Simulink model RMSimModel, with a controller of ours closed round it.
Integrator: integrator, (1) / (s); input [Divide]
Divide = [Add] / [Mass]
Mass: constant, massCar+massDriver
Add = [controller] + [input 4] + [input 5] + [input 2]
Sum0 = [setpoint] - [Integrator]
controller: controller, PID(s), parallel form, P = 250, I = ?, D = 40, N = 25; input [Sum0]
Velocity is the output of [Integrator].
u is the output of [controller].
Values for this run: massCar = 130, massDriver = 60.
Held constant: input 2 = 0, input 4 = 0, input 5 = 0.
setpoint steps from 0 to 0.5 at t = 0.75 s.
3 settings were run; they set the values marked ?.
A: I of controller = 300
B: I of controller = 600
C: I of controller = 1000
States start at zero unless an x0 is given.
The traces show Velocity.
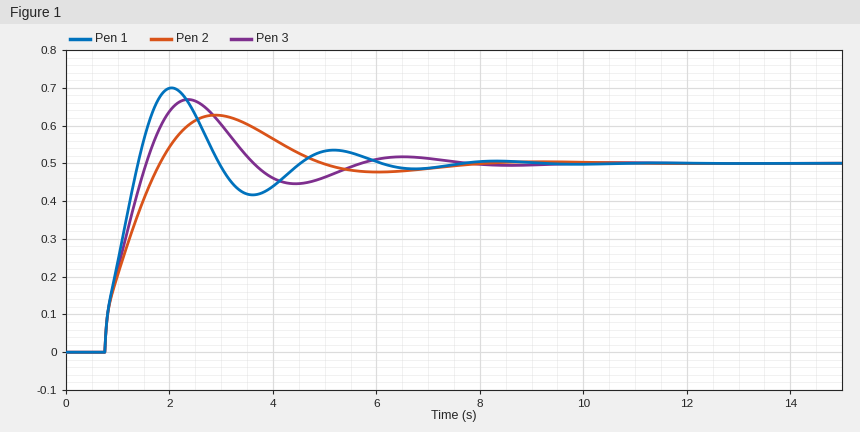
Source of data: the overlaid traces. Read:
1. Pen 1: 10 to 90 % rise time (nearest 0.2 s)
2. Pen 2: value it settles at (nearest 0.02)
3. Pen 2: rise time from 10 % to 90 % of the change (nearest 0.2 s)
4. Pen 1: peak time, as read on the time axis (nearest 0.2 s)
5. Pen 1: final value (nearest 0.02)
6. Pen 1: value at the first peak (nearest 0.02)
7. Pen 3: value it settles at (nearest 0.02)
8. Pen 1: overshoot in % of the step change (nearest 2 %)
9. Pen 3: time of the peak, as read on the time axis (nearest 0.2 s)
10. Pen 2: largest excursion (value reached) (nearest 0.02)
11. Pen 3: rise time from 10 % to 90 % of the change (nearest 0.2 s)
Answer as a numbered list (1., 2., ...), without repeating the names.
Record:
1. 0.6 s
2. 0.50
3. 0.8 s
4. 2.0 s
5. 0.50
6. 0.70
7. 0.50
8. 40 %
9. 2.4 s
10. 0.62
11. 0.6 s
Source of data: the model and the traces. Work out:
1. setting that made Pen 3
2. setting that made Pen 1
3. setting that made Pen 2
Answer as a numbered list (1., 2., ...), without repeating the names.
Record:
1. B
2. C
3. A
